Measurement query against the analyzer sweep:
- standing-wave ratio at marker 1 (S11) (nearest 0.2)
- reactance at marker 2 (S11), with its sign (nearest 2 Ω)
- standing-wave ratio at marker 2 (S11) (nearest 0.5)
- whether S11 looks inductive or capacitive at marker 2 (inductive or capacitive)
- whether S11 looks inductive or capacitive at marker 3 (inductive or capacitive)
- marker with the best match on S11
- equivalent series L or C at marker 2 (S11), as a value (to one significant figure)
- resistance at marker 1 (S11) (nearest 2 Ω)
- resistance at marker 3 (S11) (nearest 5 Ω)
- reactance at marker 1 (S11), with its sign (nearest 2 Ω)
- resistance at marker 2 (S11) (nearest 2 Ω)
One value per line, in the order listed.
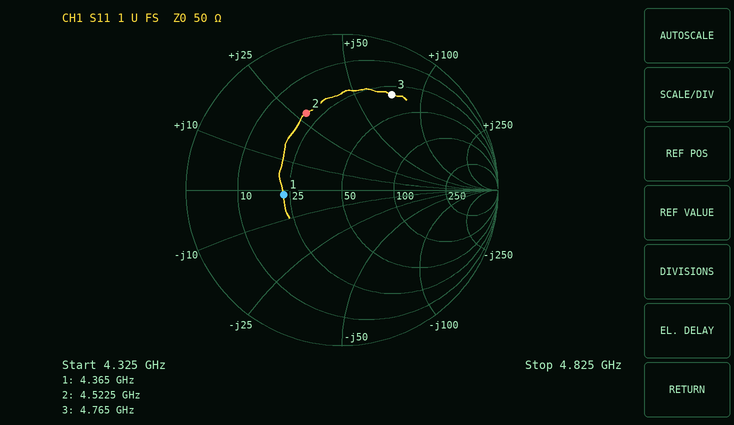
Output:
2.2
+28 Ω
3.5
inductive
inductive
marker 1
1.0 nH
22 Ω
30 Ω
-2 Ω
20 Ω
